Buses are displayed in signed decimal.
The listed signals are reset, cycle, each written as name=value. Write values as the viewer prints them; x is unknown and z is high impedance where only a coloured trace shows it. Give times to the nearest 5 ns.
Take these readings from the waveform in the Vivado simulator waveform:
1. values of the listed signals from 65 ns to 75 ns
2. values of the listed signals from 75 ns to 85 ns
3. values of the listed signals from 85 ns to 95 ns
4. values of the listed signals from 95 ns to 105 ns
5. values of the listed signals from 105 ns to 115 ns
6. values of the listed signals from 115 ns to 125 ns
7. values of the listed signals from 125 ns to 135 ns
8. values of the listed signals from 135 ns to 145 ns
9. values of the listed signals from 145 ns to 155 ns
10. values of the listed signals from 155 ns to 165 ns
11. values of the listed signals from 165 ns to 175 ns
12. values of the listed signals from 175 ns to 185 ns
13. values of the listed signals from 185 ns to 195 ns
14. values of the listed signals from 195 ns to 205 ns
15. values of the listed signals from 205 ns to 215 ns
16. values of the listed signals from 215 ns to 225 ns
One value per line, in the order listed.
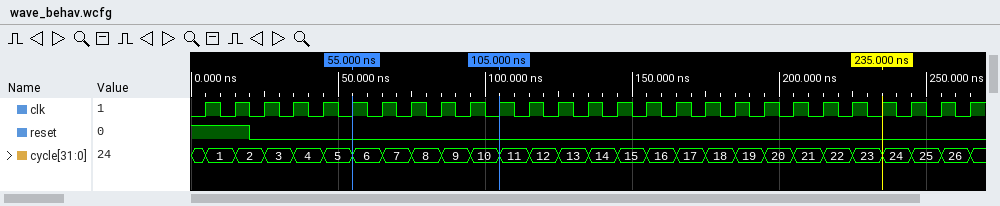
reset=0, cycle=7
reset=0, cycle=8
reset=0, cycle=9
reset=0, cycle=10
reset=0, cycle=11
reset=0, cycle=12
reset=0, cycle=13
reset=0, cycle=14
reset=0, cycle=15
reset=0, cycle=16
reset=0, cycle=17
reset=0, cycle=18
reset=0, cycle=19
reset=0, cycle=20
reset=0, cycle=21
reset=0, cycle=22
